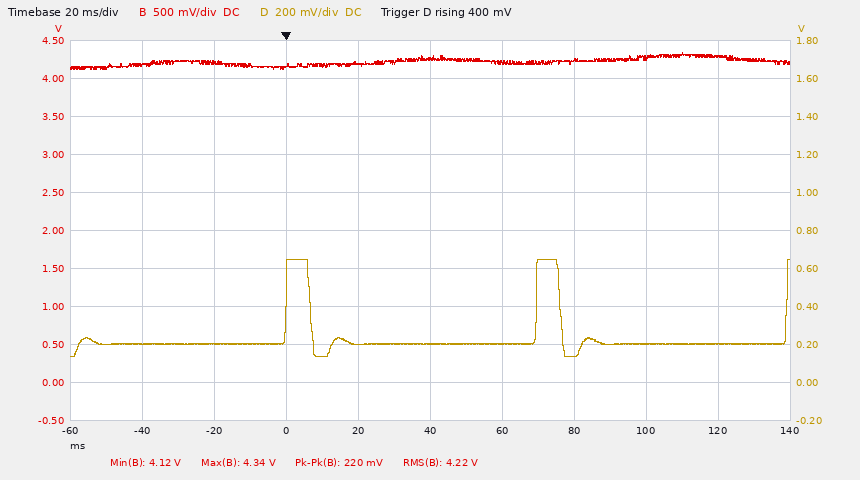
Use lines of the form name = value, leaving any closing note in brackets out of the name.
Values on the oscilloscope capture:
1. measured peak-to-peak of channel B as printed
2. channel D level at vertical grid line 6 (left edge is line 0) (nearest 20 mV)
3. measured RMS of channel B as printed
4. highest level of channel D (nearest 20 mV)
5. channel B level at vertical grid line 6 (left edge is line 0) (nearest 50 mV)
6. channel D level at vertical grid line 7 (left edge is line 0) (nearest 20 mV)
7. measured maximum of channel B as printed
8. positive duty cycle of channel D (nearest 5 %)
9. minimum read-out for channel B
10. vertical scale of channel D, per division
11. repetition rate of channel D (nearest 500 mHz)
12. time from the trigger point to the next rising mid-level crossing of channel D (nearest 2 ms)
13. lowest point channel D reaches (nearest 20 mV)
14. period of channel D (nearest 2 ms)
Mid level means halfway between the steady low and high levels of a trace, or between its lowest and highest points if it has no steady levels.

measured peak-to-peak of channel B as printed = 220 mV
channel D level at vertical grid line 6 (left edge is line 0) = 200 mV
measured RMS of channel B as printed = 4.22 V
highest level of channel D = 640 mV
channel B level at vertical grid line 6 (left edge is line 0) = 4.20 V
channel D level at vertical grid line 7 (left edge is line 0) = 140 mV
measured maximum of channel B as printed = 4.34 V
positive duty cycle of channel D = 10 %
minimum read-out for channel B = 4.12 V
vertical scale of channel D, per division = 200 mV
repetition rate of channel D = 14.5 Hz
time from the trigger point to the next rising mid-level crossing of channel D = 70 ms
lowest point channel D reaches = 140 mV
period of channel D = 70 ms
